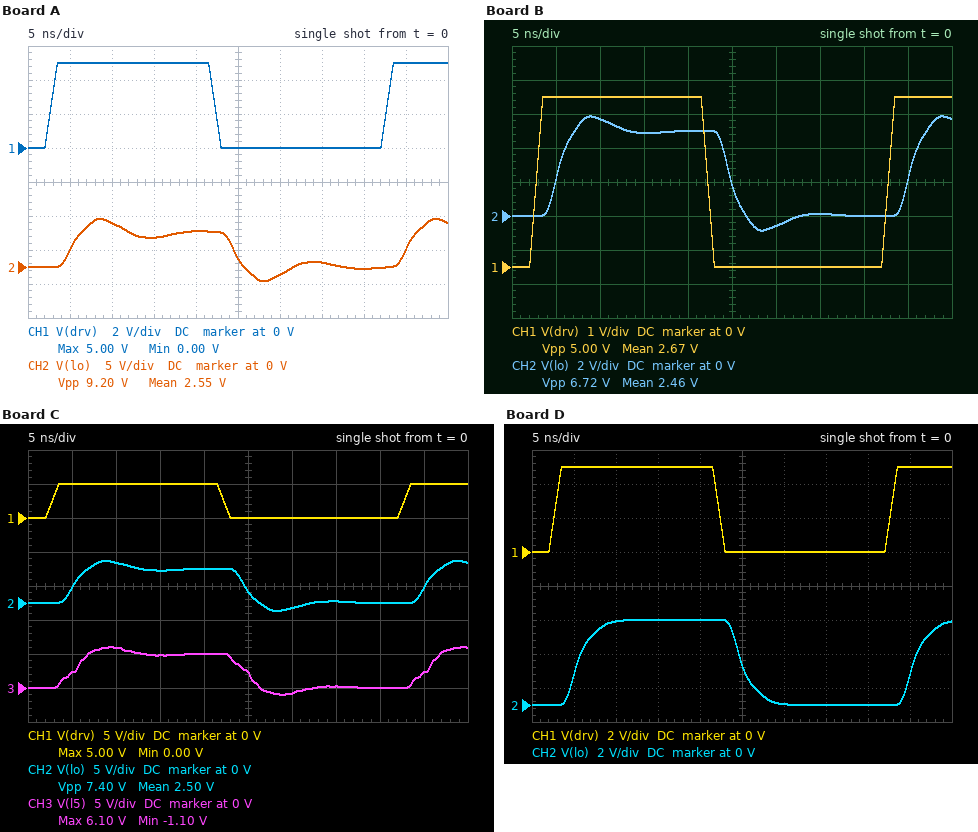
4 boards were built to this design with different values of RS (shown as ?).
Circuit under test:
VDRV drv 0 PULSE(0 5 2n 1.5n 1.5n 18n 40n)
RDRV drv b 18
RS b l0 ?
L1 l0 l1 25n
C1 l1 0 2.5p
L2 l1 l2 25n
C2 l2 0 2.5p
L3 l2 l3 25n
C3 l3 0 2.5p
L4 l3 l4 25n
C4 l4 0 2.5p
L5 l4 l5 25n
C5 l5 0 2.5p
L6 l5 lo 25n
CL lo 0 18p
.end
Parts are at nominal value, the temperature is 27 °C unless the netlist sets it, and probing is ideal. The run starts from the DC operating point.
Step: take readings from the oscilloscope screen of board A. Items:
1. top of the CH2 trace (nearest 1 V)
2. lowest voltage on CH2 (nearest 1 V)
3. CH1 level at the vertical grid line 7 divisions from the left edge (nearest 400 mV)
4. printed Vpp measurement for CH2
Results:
7 V
-2 V
0 V
9.20 V
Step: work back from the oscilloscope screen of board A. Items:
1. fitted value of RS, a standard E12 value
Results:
22 Ω
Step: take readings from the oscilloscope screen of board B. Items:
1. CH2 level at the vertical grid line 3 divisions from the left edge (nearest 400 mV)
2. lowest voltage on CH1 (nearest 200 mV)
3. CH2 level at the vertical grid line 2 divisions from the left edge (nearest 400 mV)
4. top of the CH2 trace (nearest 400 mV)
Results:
4.8 V
0 V
5.6 V
6.0 V
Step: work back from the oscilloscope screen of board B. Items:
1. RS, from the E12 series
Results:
47 Ω
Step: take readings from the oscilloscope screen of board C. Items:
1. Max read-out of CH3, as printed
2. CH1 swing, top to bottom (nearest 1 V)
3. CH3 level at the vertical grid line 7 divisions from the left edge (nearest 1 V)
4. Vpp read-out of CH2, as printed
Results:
6.10 V
5 V
0 V
7.40 V
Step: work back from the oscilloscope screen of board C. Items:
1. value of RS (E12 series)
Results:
39 Ω
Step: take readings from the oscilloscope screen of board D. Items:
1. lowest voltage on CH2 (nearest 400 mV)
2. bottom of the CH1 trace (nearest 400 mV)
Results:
0 V
0 V
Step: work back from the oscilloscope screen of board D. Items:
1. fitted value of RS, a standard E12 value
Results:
82 Ω
